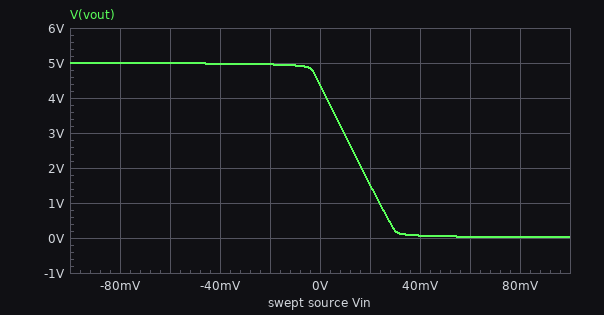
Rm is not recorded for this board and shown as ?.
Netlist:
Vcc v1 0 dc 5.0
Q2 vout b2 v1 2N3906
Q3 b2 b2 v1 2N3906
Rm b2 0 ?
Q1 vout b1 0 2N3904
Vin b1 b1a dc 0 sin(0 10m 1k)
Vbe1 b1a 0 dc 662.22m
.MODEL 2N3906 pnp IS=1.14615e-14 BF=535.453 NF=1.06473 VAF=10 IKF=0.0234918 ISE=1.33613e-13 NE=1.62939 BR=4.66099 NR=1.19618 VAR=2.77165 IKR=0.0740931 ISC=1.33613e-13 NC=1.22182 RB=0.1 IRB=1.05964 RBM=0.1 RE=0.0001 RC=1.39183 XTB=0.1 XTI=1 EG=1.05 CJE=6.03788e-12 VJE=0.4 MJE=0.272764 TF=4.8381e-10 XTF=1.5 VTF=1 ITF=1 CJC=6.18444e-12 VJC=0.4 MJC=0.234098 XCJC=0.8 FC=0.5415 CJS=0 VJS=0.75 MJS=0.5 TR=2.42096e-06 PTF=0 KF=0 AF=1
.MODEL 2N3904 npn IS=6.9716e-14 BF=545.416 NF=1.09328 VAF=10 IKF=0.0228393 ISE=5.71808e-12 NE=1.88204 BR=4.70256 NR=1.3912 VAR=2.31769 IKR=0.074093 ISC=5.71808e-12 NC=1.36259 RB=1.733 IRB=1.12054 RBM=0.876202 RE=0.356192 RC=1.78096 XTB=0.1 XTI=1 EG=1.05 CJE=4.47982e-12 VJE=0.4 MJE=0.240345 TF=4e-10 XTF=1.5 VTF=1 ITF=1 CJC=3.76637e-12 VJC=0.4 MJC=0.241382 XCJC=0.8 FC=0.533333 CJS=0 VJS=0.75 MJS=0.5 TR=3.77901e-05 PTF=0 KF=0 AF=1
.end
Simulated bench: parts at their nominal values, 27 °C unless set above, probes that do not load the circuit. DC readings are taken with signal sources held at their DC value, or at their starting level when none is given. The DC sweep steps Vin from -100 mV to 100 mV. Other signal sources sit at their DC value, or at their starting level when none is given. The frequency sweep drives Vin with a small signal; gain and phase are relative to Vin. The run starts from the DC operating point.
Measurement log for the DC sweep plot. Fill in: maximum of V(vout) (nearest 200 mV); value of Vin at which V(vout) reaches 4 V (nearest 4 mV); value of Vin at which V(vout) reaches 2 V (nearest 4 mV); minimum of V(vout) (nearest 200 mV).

5.0 V
4 mV
16 mV
0 V
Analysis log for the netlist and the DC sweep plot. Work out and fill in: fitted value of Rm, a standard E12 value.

3.9 kΩ
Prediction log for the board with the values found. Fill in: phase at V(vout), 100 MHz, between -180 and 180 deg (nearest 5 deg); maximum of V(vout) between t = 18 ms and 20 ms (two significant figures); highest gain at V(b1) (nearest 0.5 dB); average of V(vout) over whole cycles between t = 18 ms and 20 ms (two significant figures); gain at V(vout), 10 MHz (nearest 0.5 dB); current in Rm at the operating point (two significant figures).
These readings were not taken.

105 deg
4.9 V
0 dB
4.2 V
30.5 dB
1.1 mA
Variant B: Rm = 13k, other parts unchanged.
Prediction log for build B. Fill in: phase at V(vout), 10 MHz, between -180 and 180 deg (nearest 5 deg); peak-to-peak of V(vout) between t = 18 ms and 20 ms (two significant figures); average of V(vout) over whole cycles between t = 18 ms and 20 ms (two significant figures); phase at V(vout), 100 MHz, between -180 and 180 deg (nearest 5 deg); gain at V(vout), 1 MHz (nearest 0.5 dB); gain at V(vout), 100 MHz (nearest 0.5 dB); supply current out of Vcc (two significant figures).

15 deg
490 mV
150 mV
0 deg
7.0 dB
-0.5 dB
850 µA
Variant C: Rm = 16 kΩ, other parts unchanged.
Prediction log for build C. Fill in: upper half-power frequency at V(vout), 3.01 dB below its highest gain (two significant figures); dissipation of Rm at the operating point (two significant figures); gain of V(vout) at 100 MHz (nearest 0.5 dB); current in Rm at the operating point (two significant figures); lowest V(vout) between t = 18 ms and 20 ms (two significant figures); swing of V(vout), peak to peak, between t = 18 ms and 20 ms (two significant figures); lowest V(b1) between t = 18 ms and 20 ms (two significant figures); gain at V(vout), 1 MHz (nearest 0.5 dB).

640 kHz
1.2 mW
-0.5 dB
270 µA
32 mV
61 mV
650 mV
2.5 dB
